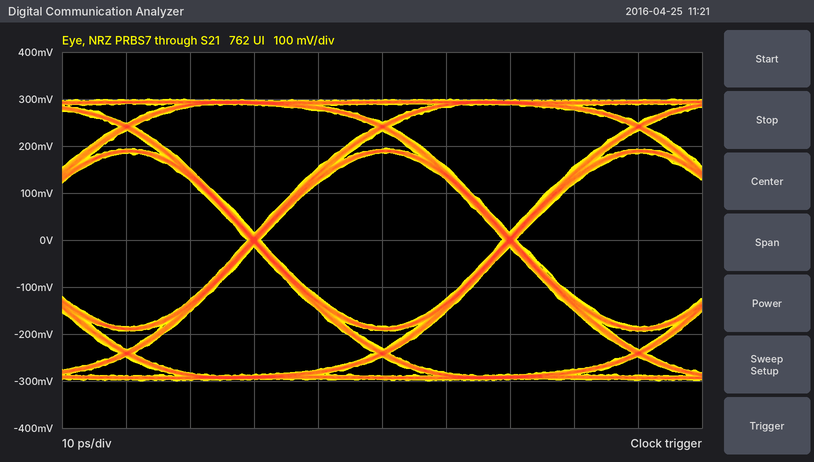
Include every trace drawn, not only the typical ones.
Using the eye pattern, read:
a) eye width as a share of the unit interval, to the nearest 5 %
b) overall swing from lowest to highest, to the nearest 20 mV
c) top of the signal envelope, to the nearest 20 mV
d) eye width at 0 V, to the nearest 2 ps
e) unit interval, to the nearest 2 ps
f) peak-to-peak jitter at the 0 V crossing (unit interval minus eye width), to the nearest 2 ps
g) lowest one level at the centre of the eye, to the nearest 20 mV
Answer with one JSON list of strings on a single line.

["95 %", "600 mV", "300 mV", "38 ps", "40 ps", "2 ps", "180 mV"]
